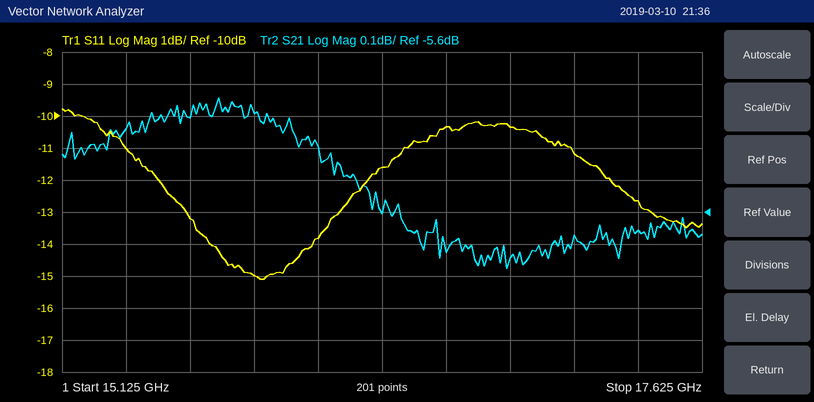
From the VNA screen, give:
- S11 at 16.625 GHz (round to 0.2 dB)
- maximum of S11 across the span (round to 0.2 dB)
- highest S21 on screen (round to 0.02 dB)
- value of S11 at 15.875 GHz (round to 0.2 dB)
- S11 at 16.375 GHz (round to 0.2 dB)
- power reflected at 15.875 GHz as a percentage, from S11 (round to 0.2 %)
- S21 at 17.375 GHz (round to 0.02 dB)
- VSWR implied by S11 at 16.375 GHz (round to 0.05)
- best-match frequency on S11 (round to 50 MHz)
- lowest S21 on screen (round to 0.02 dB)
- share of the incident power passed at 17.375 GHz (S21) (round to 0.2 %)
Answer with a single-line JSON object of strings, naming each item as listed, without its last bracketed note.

{"S11 at 16.625 GHz": "-10.4 dB", "maximum of S11 across the span": "-9.8 dB", "highest S21 on screen": "-5.24 dB", "value of S11 at 15.875 GHz": "-15.0 dB", "S11 at 16.375 GHz": "-11.6 dB", "power reflected at 15.875 GHz as a percentage, from S11": "3.2 %", "S21 at 17.375 GHz": "-5.66 dB", "VSWR implied by S11 at 16.375 GHz": "1.70", "best-match frequency on S11": "15.90 GHz", "lowest S21 on screen": "-5.78 dB", "share of the incident power passed at 17.375 GHz (S21)": "27.2 %"}
